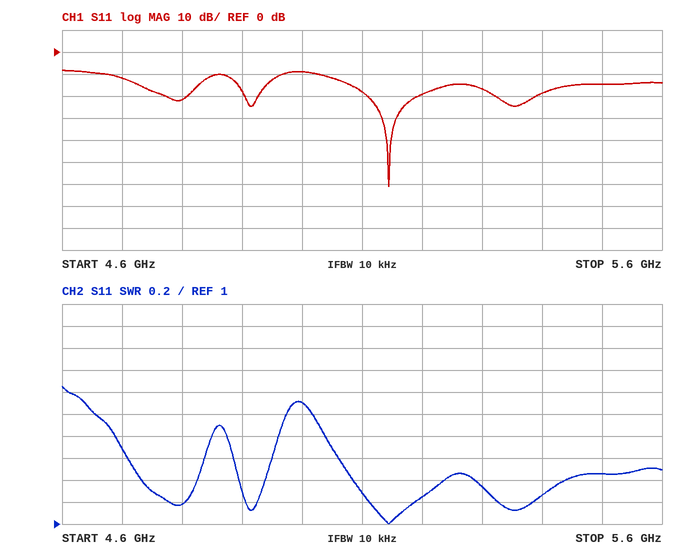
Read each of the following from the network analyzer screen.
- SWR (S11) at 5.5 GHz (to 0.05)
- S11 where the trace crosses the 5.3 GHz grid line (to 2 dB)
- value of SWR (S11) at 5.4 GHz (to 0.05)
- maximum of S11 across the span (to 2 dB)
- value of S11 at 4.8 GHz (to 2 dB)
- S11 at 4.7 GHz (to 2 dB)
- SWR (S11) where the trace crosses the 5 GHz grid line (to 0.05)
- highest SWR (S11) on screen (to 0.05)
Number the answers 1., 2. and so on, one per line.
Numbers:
1. 1.45
2. -16 dB
3. 1.25
4. -8 dB
5. -22 dB
6. -12 dB
7. 2.10
8. 2.25
